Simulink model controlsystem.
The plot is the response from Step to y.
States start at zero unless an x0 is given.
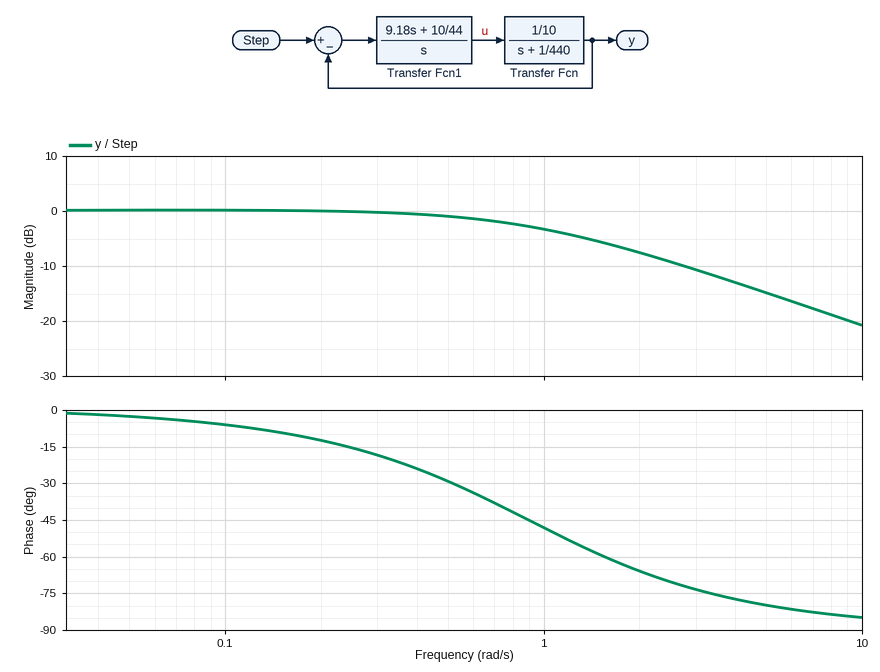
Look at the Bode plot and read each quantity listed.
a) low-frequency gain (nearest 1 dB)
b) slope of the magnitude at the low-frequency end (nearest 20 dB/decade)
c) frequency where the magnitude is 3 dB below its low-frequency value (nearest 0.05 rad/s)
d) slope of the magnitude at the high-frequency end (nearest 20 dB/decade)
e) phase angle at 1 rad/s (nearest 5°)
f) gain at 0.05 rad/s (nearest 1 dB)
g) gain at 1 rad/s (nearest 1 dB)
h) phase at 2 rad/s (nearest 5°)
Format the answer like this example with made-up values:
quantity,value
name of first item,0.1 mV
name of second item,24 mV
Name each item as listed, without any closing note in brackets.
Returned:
quantity,value
low-frequency gain,0 dB
slope of the magnitude at the low-frequency end,0 dB/decade
frequency where the magnitude is 3 dB below its low-frequency value,0.90 rad/s
slope of the magnitude at the high-frequency end,-20 dB/decade
phase angle at 1 rad/s,-50°
gain at 0.05 rad/s,0 dB
gain at 1 rad/s,-3 dB
phase at 2 rad/s,-65°
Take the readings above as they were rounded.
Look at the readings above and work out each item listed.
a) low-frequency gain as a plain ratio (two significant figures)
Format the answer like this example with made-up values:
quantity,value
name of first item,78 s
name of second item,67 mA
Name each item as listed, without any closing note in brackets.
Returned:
quantity,value
low-frequency gain as a plain ratio,1.0
